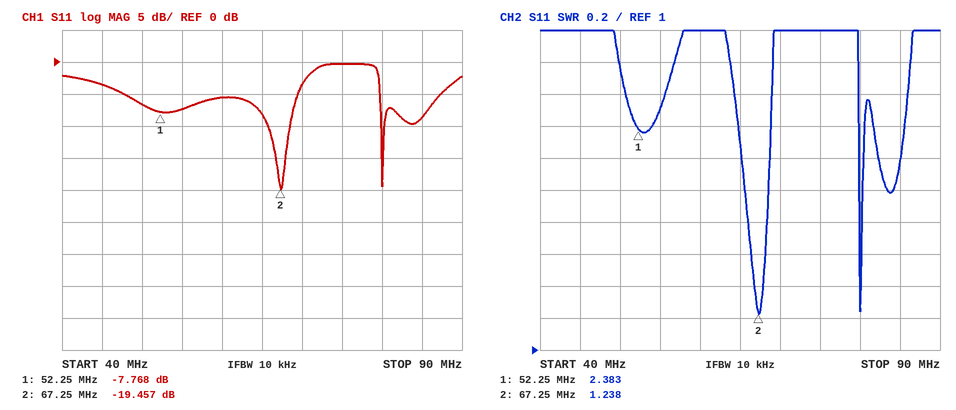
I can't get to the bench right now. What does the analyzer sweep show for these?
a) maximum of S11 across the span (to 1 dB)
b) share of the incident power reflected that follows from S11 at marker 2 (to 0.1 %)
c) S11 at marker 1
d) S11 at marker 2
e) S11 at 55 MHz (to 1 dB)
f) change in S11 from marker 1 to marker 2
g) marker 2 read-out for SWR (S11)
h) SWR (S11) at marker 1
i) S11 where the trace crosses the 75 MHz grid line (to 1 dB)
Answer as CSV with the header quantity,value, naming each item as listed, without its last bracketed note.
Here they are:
quantity,value
maximum of S11 across the span,0 dB
share of the incident power reflected that follows from S11 at marker 2,1.1 %
S11 at marker 1,-7.768 dB
S11 at marker 2,-19.457 dB
S11 at 55 MHz,-7 dB
change in S11 from marker 1 to marker 2,-11.689 dB
marker 2 read-out for SWR,1.238
SWR (S11) at marker 1,2.383
S11 where the trace crosses the 75 MHz grid line,0 dB
